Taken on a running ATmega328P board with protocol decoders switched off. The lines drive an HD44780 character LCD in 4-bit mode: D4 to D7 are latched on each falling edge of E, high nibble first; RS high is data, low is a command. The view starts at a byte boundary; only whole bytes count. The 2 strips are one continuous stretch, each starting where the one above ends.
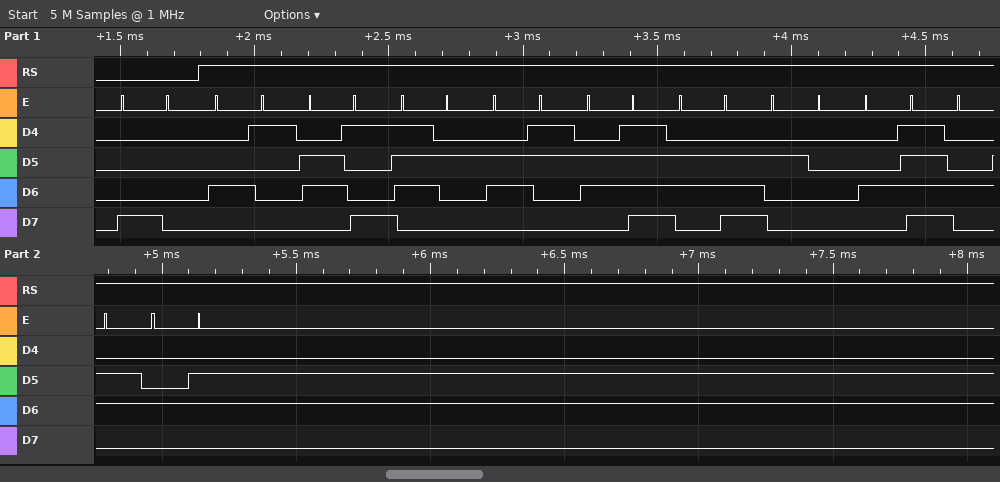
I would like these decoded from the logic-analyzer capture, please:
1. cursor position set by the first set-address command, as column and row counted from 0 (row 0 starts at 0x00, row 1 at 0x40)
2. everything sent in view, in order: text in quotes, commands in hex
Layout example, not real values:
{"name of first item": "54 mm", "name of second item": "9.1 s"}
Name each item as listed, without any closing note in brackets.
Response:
{"cursor position set by the first set-address command, as column and row counted from 0": "column 0, row 0", "everything sent in view, in order: text in quotes, commands in hex": "0x80 \"Aircon OFF\""}
